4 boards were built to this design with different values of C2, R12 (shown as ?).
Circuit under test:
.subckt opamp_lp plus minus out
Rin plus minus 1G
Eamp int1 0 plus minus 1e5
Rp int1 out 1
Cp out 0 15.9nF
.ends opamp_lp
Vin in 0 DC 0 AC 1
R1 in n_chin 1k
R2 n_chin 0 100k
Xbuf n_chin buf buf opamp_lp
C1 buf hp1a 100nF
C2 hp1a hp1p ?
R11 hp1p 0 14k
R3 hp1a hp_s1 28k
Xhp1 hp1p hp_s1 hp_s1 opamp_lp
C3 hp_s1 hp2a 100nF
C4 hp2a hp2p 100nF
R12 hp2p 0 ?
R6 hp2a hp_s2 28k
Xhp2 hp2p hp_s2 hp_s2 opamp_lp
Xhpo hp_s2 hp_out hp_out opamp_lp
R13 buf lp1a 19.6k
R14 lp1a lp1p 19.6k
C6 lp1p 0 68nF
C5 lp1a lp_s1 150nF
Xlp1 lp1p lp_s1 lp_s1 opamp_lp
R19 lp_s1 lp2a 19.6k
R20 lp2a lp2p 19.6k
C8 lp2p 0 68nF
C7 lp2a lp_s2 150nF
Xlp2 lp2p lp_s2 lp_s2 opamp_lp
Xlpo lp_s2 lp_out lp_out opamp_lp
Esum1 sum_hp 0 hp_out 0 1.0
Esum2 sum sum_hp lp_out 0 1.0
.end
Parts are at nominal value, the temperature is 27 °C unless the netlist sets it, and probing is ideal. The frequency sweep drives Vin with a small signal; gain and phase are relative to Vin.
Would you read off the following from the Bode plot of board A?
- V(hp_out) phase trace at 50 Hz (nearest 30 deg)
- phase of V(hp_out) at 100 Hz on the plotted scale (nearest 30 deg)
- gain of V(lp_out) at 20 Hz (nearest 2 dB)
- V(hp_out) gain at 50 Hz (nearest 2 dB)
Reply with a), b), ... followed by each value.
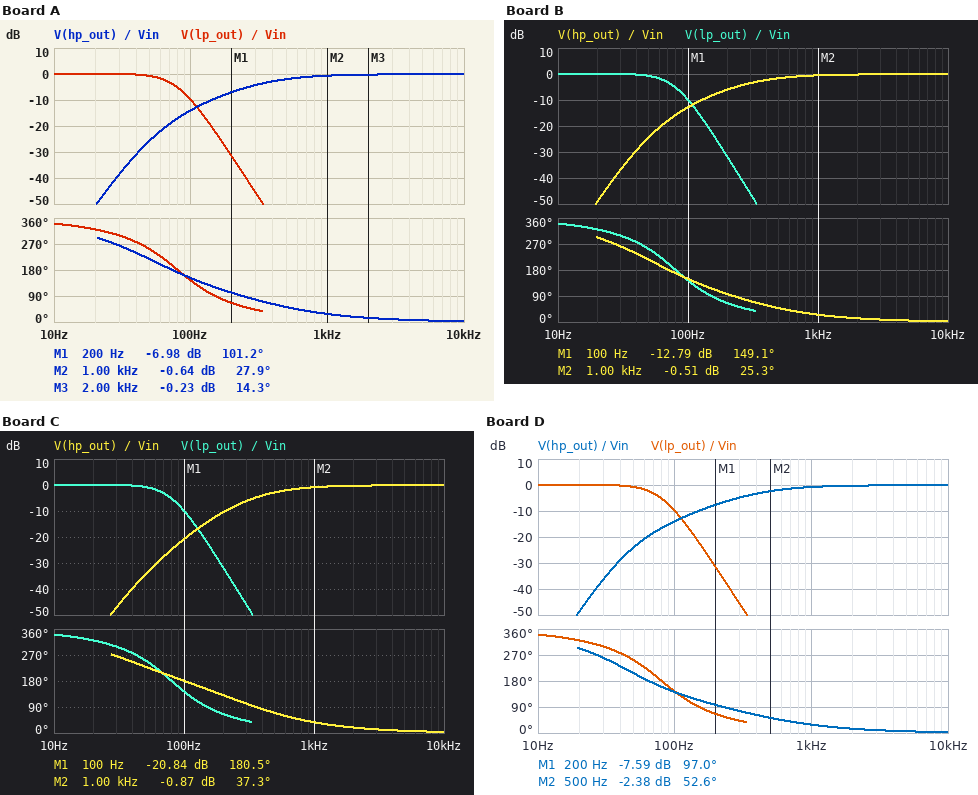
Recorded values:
a) 210 deg
b) 150 deg
c) 0 dB
d) -26 dB
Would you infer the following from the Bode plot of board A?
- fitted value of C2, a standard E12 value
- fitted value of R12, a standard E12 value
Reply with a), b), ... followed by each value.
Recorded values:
a) 39 nF
b) 33 kΩ
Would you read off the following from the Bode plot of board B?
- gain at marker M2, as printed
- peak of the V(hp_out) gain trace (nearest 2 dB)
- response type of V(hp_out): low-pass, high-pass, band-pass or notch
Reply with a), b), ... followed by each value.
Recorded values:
a) -0.51 dB
b) 0 dB
c) high-pass
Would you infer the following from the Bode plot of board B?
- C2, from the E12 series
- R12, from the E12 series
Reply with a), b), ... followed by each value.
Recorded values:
a) 47 nF
b) 33 kΩ
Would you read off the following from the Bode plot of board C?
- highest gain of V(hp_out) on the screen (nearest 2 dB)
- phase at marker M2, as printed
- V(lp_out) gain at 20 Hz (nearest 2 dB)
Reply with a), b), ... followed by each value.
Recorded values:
a) 0 dB
b) 37.3 deg
c) 0 dB
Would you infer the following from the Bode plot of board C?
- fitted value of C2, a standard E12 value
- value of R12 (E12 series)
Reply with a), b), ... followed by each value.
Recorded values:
a) 68 nF
b) 8.2 kΩ
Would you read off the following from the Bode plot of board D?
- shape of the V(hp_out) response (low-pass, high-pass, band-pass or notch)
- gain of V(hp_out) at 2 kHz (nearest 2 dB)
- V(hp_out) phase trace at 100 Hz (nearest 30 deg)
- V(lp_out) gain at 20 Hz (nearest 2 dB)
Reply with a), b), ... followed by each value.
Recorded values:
a) high-pass
b) 0 dB
c) 150 deg
d) 0 dB
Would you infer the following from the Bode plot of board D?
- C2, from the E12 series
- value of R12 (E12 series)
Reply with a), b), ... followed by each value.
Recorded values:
a) 33 nF
b) 47 kΩ
